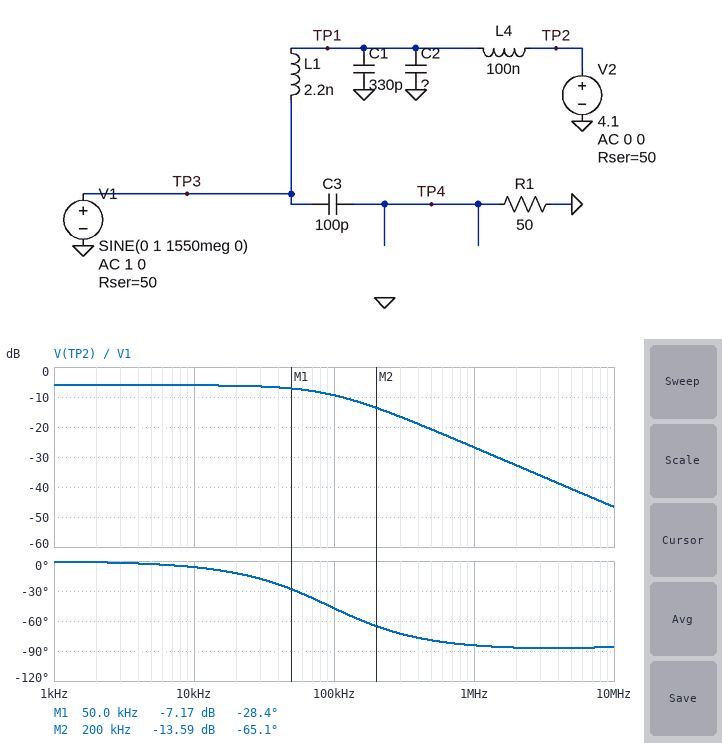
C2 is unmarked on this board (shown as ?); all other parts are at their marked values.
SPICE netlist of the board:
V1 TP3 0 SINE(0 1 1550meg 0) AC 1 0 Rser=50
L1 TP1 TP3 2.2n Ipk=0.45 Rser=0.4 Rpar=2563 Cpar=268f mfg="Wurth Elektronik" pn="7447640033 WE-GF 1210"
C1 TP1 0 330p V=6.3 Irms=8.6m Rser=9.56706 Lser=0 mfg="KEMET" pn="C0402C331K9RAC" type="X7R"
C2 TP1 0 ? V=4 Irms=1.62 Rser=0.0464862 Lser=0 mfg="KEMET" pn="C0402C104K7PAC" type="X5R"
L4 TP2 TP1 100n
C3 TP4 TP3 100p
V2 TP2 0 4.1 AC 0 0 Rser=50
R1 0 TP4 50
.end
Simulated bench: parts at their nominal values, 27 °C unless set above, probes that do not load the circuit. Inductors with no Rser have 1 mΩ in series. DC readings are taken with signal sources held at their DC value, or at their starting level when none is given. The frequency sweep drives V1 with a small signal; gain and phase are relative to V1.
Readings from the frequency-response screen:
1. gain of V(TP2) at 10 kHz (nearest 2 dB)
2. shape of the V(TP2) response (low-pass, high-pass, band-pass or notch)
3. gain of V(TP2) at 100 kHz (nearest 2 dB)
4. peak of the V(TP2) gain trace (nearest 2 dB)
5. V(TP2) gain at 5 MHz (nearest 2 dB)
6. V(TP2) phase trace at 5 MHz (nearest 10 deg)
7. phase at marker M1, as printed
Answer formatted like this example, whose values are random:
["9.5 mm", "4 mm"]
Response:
["-6 dB", "low-pass", "-10 dB", "-6 dB", "-40 dB", "-90 deg", "-28.4 deg"]
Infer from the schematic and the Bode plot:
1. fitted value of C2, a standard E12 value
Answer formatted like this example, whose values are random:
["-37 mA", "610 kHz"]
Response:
["68 nF"]
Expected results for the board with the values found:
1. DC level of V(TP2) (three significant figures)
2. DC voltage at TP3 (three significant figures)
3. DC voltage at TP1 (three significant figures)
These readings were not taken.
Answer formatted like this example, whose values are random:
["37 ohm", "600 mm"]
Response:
["2.06 V", "2.04 V", "2.06 V"]
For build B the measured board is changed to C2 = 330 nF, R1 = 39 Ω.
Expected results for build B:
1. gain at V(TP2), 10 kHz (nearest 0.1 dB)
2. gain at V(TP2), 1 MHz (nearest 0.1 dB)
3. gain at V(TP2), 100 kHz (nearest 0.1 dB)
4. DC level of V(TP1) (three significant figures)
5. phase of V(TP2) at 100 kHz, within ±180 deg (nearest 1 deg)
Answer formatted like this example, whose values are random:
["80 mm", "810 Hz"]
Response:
["-7.1 dB", "-40.4 dB", "-20.6 dB", "2.06 V", "-79 deg"]
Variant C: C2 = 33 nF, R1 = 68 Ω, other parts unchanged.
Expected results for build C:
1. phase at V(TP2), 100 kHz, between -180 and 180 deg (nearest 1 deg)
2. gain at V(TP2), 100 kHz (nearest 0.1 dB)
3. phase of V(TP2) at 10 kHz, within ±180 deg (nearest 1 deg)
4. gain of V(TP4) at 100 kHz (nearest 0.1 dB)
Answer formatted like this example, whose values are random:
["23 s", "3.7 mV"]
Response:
["-28 deg", "-7.1 dB", "-3 deg", "-54.4 dB"]
